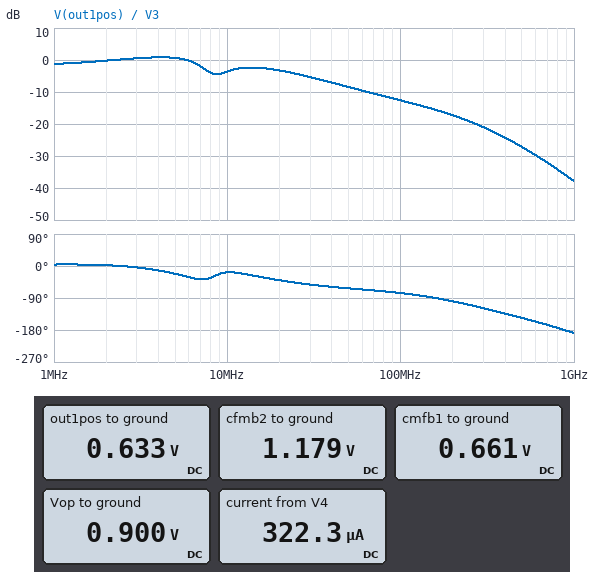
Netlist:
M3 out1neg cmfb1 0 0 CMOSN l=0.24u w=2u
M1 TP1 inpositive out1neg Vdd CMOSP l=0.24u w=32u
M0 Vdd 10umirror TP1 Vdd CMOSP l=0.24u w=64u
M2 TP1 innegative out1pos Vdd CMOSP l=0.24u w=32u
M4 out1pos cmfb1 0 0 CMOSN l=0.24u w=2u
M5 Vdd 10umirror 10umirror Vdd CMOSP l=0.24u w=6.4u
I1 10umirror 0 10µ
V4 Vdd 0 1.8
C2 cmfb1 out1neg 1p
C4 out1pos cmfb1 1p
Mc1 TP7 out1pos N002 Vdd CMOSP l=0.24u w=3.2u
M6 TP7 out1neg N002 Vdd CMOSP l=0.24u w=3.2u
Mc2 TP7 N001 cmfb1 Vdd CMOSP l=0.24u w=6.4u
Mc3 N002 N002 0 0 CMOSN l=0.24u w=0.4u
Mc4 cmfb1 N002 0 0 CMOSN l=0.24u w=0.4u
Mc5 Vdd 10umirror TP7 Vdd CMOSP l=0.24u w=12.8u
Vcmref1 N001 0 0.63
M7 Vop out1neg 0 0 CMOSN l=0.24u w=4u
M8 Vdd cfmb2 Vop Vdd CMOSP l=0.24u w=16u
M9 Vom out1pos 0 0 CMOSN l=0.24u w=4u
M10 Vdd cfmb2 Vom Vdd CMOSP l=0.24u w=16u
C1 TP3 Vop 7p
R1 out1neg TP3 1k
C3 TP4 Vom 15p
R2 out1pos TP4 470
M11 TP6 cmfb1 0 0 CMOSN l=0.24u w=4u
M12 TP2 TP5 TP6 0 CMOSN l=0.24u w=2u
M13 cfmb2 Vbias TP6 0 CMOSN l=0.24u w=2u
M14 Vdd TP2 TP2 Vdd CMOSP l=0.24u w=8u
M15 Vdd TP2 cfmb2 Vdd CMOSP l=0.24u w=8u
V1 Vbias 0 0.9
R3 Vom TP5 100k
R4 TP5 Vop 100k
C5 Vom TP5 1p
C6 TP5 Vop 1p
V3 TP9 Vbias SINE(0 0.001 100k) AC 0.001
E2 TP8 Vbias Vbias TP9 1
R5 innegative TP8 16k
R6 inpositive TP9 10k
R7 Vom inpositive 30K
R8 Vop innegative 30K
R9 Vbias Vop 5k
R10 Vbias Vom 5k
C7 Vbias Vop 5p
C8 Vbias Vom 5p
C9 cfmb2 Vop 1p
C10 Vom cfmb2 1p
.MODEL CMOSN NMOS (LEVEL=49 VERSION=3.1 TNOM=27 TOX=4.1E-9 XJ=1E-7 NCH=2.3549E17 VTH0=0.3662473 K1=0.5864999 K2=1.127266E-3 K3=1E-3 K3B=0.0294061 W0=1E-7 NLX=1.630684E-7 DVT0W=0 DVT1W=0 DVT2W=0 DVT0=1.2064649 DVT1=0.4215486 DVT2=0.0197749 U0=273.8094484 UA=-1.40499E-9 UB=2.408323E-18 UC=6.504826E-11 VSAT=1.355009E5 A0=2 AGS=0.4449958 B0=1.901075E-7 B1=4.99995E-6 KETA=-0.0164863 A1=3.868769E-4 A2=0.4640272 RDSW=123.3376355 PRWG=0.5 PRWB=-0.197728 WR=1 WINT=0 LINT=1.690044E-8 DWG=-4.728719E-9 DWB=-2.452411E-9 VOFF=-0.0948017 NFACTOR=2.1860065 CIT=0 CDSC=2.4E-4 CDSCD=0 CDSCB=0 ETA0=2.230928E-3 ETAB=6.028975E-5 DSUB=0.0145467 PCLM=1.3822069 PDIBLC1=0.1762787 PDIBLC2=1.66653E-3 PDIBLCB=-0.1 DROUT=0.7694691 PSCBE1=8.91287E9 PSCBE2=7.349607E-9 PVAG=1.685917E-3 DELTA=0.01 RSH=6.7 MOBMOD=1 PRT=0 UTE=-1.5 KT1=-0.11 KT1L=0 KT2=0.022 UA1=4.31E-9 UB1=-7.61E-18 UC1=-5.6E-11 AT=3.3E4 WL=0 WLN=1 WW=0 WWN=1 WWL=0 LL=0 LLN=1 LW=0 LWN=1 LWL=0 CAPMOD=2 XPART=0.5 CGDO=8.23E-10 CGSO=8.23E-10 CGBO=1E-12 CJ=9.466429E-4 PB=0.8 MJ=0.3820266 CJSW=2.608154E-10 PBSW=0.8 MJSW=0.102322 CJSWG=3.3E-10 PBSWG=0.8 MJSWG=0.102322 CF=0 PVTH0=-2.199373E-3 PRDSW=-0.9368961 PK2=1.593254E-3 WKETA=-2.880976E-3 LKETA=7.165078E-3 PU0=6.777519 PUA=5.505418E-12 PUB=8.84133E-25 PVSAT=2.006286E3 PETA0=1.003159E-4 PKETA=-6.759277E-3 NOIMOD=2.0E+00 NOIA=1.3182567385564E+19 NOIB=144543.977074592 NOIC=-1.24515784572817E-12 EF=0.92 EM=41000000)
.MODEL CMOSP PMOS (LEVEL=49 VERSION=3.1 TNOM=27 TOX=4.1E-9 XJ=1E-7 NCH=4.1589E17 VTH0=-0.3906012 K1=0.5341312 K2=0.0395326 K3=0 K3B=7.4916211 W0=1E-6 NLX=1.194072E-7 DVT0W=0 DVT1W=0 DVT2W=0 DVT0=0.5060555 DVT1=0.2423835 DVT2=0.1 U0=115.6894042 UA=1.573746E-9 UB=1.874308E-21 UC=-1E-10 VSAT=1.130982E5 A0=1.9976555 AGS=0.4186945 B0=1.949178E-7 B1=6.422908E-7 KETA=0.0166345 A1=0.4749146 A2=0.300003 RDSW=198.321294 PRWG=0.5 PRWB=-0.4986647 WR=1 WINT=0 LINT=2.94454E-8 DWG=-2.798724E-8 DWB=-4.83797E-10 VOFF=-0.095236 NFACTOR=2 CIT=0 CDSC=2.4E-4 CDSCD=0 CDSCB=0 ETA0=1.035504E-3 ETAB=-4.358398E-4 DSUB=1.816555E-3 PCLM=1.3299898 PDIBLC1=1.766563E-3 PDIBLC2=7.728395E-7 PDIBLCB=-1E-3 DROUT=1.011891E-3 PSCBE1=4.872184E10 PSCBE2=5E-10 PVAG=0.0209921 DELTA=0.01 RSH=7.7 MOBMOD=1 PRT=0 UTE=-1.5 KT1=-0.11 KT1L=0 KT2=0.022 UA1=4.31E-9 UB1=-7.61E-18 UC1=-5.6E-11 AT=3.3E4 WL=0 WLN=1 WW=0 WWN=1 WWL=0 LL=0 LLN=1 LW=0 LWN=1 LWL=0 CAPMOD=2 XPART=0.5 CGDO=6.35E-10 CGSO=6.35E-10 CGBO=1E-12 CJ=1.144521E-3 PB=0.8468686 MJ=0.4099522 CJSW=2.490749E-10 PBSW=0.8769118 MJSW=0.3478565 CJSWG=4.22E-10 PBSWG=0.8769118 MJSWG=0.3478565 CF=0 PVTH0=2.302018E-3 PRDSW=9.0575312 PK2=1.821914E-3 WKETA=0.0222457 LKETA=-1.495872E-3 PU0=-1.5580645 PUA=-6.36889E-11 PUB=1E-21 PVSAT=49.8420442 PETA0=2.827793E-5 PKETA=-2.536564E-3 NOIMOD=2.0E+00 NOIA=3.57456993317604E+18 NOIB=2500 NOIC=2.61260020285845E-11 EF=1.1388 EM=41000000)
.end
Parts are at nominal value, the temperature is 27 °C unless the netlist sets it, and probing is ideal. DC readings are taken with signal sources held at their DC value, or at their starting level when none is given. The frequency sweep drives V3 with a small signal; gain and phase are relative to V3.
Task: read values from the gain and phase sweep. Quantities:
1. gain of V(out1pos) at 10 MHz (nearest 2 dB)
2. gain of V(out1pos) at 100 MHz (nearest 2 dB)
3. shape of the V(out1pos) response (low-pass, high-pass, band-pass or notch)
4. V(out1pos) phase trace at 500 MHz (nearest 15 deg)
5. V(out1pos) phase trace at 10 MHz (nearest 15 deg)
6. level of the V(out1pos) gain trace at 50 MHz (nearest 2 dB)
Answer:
-4 dB
-12 dB
low-pass
-150 deg
-15 deg
-8 dB
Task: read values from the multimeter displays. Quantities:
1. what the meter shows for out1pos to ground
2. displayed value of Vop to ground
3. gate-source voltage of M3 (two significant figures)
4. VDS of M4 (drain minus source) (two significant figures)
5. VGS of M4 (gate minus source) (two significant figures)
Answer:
0.633 V
0.900 V
660 mV
630 mV
660 mV
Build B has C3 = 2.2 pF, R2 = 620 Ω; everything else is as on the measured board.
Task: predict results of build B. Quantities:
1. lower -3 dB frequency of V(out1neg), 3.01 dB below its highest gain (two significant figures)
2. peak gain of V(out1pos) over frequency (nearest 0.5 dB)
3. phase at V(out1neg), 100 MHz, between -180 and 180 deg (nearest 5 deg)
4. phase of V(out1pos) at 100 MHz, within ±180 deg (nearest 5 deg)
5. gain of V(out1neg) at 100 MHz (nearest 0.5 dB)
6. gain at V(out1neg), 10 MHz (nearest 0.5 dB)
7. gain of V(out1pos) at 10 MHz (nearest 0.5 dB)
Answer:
2.0 MHz
8.0 dB
110 deg
-90 deg
-10.0 dB
0 dB
5.5 dB
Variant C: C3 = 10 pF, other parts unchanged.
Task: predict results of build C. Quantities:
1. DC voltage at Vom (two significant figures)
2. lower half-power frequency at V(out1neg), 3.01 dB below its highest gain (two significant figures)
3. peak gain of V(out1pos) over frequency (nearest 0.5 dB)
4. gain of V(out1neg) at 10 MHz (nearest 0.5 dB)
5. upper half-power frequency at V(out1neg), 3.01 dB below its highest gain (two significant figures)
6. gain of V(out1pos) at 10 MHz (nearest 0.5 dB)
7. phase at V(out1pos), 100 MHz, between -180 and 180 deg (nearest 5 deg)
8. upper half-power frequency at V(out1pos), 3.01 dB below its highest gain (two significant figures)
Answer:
900 mV
2.3 MHz
1.5 dB
2.5 dB
18 MHz
-1.0 dB
-80 deg
13 MHz
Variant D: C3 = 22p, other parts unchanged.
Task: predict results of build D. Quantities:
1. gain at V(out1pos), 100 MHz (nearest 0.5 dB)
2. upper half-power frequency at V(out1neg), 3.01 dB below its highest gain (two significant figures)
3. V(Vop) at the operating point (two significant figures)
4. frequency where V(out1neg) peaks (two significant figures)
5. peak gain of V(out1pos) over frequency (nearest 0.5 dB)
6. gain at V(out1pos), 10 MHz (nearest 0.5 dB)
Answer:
-13.0 dB
15 MHz
900 mV
8.1 MHz
0 dB
-4.5 dB
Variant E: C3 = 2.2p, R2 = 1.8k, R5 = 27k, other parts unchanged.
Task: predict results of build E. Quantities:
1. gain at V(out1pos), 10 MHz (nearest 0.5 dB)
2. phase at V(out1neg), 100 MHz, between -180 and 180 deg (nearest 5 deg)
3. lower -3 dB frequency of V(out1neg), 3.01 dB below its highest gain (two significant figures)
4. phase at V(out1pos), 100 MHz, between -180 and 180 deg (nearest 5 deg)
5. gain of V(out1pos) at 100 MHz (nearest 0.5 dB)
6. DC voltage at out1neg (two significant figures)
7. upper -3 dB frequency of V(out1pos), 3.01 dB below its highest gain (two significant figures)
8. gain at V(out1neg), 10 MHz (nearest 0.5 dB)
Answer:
4.5 dB
100 deg
2.8 MHz
-85 deg
-7.0 dB
630 mV
22 MHz
-0.5 dB
